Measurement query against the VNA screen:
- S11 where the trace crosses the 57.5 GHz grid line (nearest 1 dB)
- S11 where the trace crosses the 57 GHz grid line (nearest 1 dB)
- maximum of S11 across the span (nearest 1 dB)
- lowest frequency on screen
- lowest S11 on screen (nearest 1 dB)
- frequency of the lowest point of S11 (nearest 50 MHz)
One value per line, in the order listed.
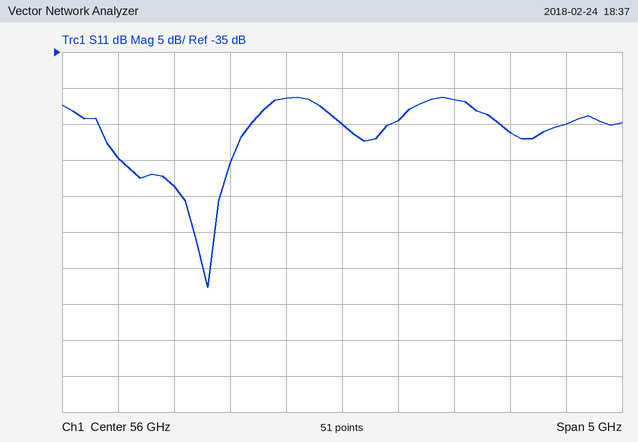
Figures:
-46 dB
-42 dB
-41 dB
53.5 GHz
-68 dB
54.80 GHz
